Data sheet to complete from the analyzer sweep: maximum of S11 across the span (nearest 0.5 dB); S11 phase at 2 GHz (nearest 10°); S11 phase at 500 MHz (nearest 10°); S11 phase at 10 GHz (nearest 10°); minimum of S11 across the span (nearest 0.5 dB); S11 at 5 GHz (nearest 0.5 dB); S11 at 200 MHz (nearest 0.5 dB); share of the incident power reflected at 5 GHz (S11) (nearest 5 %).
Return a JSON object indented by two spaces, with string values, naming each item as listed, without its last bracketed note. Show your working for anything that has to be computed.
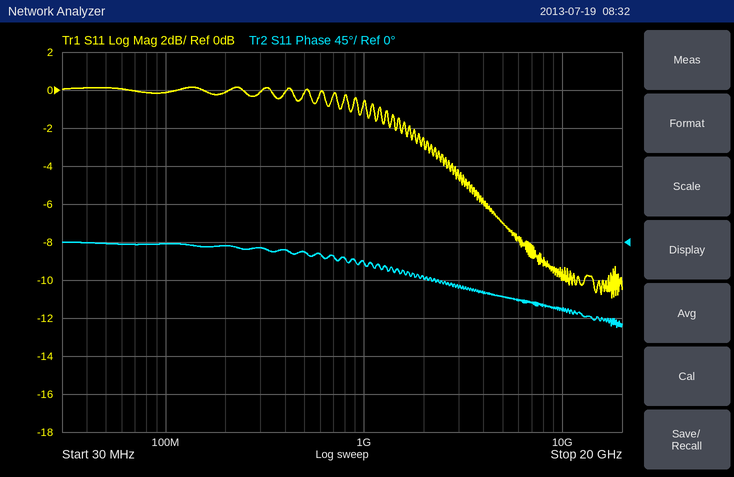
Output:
{
  "maximum of S11 across the span": "0.0 dB",
  "S11 phase at 2 GHz": "-40°",
  "S11 phase at 500 MHz": "-10°",
  "S11 phase at 10 GHz": "-80°",
  "minimum of S11 across the span": "-11.0 dB",
  "S11 at 5 GHz": "-7.0 dB",
  "S11 at 200 MHz": "0.0 dB",
  "share of the incident power reflected at 5 GHz (S11)": "10^(-7/10) ≈ 20 %"
}
